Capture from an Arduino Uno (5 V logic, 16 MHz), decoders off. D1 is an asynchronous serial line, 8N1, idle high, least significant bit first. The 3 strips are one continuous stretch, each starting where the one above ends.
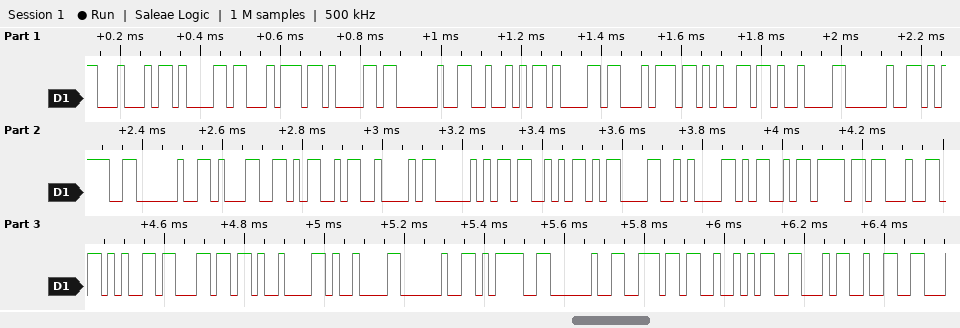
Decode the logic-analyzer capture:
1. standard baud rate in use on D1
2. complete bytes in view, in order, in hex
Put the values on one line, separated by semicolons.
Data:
57600 baud; 44 61 74 61 20 52 61 74 65 09 20 3D 20 31 4D 42 50 53 0D 0A 4D 6F 64 65 6C 09 09 20 3D 20 6E 52 46 32
